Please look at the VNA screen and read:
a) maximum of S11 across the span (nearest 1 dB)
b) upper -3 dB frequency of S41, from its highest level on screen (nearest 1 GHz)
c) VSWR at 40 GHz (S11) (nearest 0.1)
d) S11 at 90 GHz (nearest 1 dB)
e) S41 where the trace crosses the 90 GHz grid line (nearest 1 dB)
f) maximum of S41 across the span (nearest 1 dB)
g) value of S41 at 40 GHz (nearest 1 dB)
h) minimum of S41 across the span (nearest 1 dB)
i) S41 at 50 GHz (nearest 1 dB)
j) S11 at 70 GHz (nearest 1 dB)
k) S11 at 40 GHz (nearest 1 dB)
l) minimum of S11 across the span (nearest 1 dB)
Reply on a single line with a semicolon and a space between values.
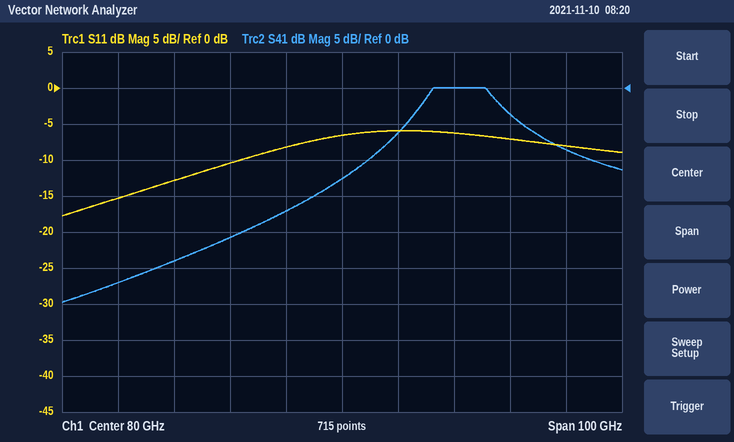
-6 dB; 109 GHz; 1.4; -6 dB; -6 dB; 0 dB; -27 dB; -30 dB; -24 dB; -8 dB; -15 dB; -18 dB
